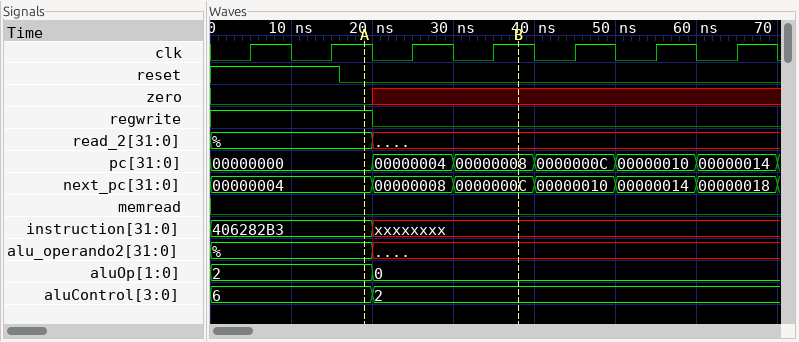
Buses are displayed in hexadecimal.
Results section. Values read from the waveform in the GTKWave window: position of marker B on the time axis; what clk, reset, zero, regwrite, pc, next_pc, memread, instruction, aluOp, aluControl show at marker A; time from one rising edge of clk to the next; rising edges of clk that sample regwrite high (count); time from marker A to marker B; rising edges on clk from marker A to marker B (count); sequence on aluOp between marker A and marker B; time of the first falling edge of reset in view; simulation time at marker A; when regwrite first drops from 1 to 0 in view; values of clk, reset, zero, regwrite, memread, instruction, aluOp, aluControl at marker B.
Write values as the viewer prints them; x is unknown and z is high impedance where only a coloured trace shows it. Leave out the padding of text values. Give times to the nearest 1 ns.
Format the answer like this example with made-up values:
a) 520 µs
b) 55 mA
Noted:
a) 38 ns
b) clk=1, reset=0, zero=0, regwrite=1, pc=00000000, next_pc=00000004, memread=0, instruction=406282B3, aluOp=2, aluControl=6
c) 10 ns
d) 2
e) 19 ns
f) 2
g) 2, 0
h) 16 ns
i) 19 ns
j) 20 ns
k) clk=1, reset=0, zero=x, regwrite=0, memread=0, instruction=xxxxxxxx, aluOp=0, aluControl=2
